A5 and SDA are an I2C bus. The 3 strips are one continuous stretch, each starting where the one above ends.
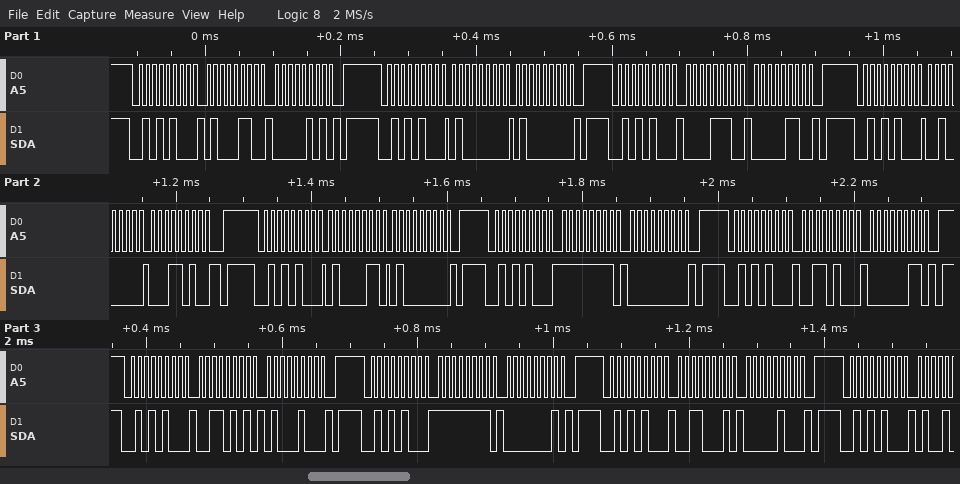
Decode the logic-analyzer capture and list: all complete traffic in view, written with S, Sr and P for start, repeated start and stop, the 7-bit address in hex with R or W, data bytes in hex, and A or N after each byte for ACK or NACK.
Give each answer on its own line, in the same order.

S 2AW A 46 A 05 A P S 2AW A 40 A 40 A P S 2AW A 0E A 06 A P S 2AW A 20 A 1A A P S 2AW A 43 A 40 A P S 2AW A FF A 00 A P S 2AW A 34 A 03 A P S 2AW A 35 A 44 A P S 2AW A FF A 01 A P S 2AW A 31 A 04 A P S 2AW A
